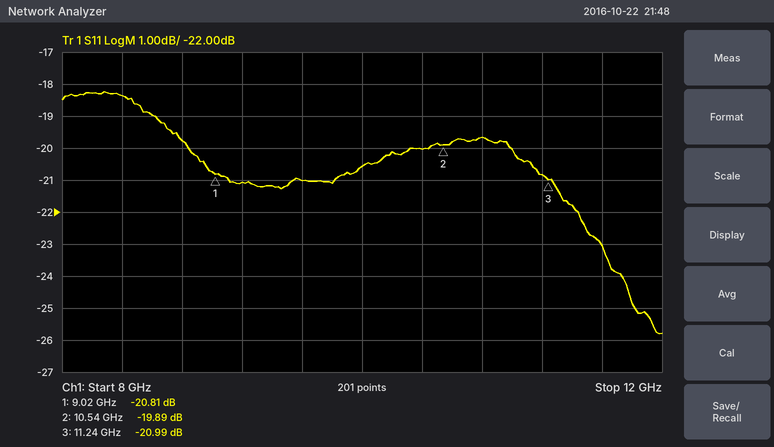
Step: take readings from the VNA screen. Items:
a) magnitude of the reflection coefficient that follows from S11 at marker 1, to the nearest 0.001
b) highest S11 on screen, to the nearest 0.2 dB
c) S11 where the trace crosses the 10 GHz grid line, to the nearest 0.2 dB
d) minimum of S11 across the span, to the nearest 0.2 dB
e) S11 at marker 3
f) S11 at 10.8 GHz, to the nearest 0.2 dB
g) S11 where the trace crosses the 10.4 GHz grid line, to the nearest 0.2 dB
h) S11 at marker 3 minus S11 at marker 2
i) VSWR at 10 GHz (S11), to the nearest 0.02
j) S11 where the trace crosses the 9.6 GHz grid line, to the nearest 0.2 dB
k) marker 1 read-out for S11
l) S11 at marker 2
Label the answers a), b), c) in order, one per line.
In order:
a) 0.091
b) -18.2 dB
c) -20.6 dB
d) -25.8 dB
e) -20.99 dB
f) -19.6 dB
g) -20.0 dB
h) -1.10 dB
i) 1.20
j) -21.0 dB
k) -20.81 dB
l) -19.89 dB
